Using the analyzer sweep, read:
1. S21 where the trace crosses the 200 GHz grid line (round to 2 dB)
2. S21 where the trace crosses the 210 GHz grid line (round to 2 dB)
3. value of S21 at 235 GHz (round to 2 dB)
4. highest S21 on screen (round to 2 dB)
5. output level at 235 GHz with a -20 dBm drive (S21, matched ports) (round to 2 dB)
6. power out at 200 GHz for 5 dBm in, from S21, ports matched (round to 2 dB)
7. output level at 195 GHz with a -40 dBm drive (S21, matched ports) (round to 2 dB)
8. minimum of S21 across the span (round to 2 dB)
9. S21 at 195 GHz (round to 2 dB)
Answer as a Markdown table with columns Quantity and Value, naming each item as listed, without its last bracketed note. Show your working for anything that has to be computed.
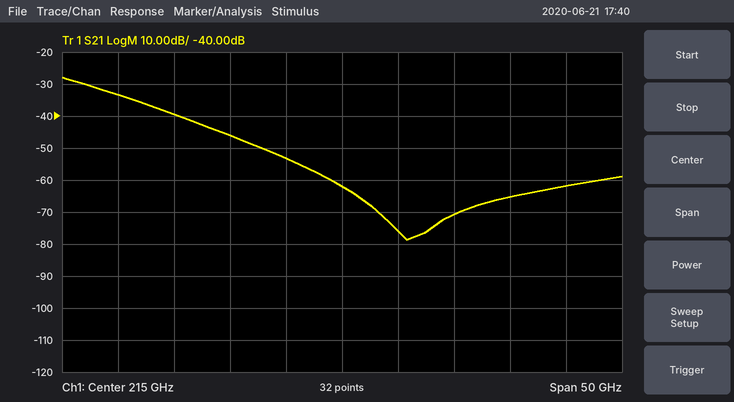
| Quantity | Value |
|---|---|
| S21 where the trace crosses the 200 GHz grid line | -40 dB |
| S21 where the trace crosses the 210 GHz grid line | -54 dB |
| value of S21 at 235 GHz | -62 dB |
| highest S21 on screen | -28 dB |
| output level at 235 GHz with a -20 dBm drive (S21, matched ports) | -20 dBm + (-62 dB) = -82 dBm |
| power out at 200 GHz for 5 dBm in, from S21, ports matched | 5 dBm + (-40 dB) = -34 dBm |
| output level at 195 GHz with a -40 dBm drive (S21, matched ports) | -40 dBm + (-34 dB) = -74 dBm |
| minimum of S21 across the span | -78 dB |
| S21 at 195 GHz | -34 dB |
